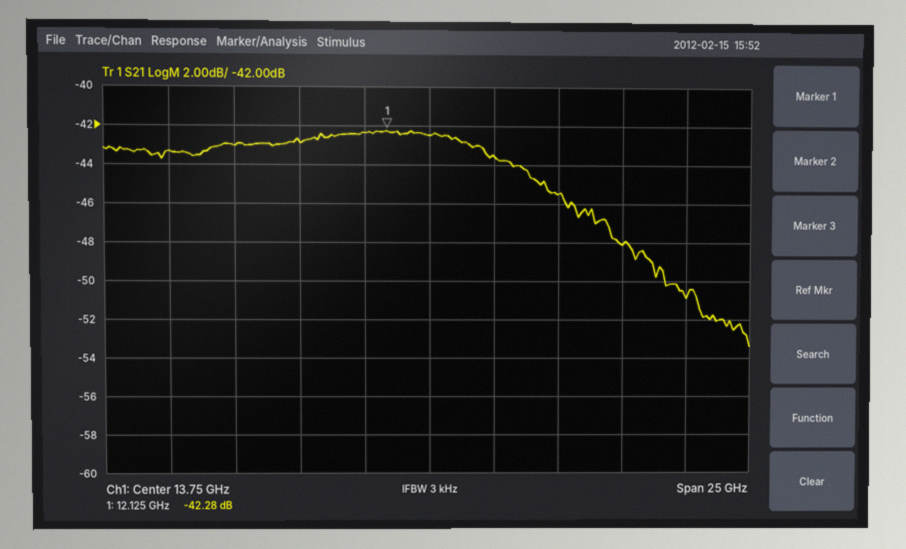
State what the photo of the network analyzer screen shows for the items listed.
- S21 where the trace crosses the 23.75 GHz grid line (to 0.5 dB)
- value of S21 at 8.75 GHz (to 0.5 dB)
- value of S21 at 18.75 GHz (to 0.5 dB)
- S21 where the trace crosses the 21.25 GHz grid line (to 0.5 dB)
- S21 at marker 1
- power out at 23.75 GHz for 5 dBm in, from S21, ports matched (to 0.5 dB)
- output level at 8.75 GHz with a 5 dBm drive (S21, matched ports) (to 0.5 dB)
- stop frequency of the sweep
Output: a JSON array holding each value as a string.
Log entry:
["-51.0 dB", "-43.0 dB", "-45.5 dB", "-48.0 dB", "-42.28 dB", "-46.0 dBm", "-38.0 dBm", "26.25 GHz"]
